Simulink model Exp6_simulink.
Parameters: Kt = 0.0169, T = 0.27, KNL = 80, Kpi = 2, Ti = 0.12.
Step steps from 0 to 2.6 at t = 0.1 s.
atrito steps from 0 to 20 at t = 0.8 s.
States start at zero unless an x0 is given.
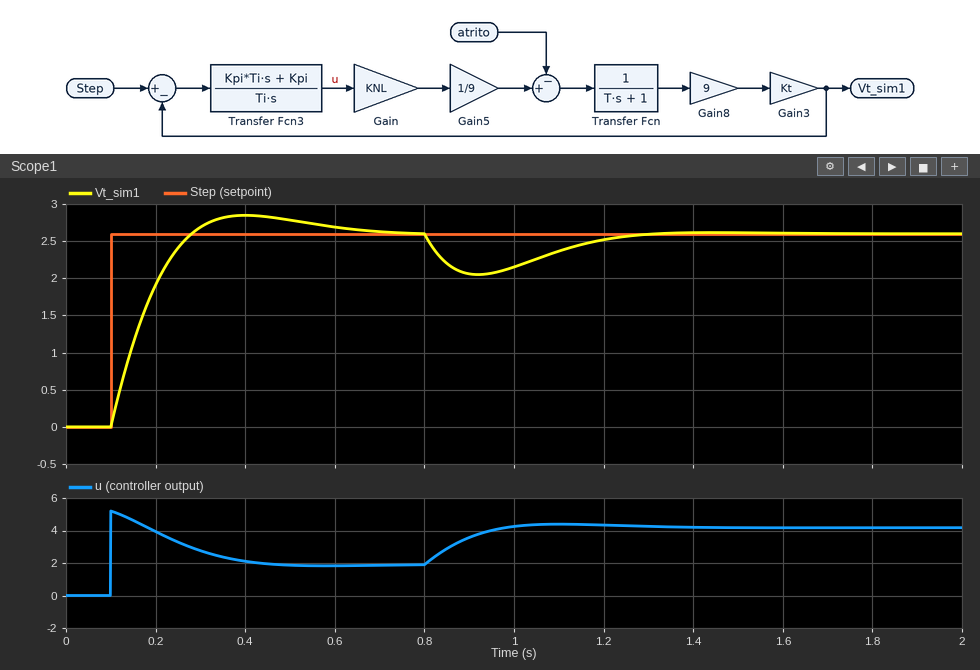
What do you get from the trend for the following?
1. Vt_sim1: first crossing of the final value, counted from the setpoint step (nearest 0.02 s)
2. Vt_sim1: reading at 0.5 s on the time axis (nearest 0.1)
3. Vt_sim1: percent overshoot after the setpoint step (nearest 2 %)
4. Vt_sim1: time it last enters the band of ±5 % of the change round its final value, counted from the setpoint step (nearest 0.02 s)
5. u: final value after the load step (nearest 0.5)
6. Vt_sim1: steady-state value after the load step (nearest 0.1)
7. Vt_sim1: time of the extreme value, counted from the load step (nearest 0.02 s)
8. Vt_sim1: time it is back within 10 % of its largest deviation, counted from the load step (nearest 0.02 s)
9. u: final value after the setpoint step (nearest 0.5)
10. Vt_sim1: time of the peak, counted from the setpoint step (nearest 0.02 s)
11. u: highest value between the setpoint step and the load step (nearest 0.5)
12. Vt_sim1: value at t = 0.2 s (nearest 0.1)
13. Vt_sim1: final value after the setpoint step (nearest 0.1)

0.18 s
2.8
10 %
0.46 s
4.0
2.6
0.12 s
0.42 s
2.0
0.30 s
5.0
1.9
2.6
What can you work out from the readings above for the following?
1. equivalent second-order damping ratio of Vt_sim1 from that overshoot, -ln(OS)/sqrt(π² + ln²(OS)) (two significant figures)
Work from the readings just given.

0.59
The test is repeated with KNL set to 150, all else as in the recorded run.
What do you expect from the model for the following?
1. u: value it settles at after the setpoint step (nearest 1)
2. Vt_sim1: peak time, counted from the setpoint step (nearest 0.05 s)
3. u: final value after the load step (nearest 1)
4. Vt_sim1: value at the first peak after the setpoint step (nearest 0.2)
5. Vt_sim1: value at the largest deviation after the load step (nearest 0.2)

1
0.20 s
2
2.8
2.2
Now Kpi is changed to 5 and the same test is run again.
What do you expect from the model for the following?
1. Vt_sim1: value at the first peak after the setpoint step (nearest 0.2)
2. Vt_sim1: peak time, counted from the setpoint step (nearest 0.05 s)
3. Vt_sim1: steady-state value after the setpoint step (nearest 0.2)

2.8
0.15 s
2.6
